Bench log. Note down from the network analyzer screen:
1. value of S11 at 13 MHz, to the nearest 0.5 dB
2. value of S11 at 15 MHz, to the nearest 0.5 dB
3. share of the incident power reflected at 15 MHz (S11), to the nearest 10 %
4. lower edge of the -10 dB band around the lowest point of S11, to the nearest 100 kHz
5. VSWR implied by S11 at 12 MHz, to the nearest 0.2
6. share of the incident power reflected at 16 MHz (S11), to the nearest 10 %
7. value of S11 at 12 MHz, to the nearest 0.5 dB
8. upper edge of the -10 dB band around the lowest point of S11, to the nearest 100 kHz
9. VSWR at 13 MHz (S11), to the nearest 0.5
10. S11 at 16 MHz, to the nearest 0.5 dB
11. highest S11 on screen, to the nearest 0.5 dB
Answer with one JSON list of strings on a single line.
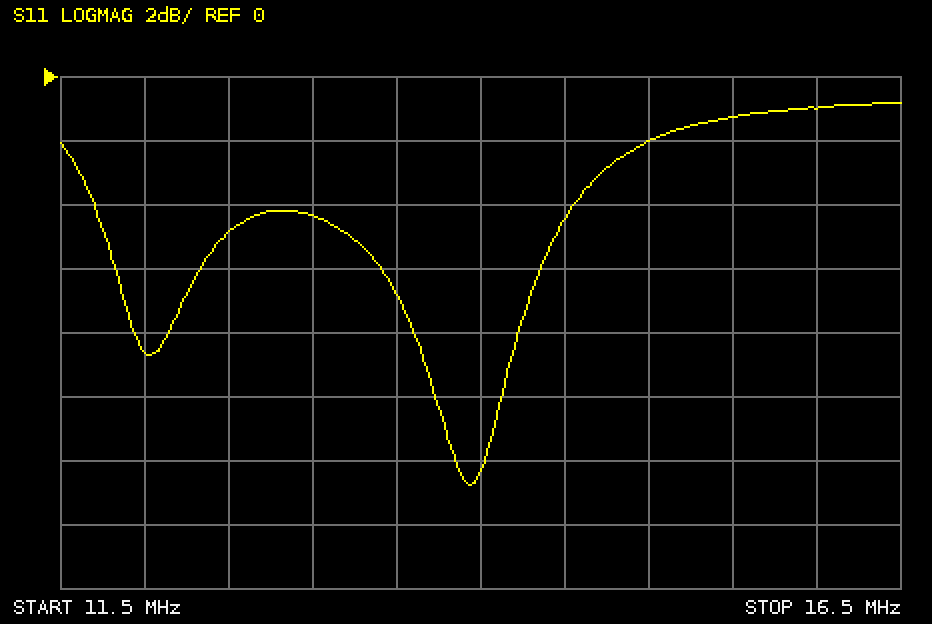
["-4.5 dB", "-2.0 dB", "60 %", "13.7 MHz", "2.2", "80 %", "-8.5 dB", "14.1 MHz", "4.0", "-1.0 dB", "-1.0 dB"]
